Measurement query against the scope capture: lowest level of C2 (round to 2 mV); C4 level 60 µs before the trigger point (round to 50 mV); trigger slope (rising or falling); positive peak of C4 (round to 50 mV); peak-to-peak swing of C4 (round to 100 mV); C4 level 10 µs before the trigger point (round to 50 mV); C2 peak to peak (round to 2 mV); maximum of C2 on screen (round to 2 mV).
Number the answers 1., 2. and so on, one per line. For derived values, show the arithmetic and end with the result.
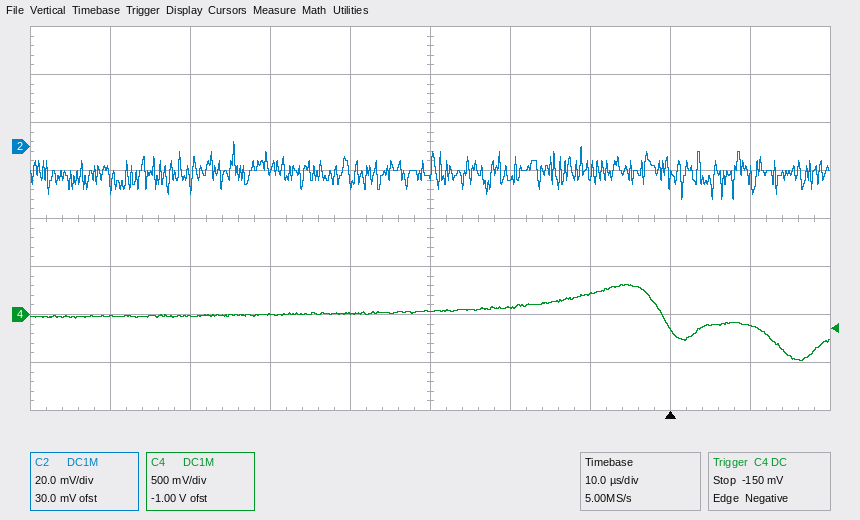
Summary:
1. -22 mV
2. 0 mV
3. falling
4. 300 mV
5. 800 mV
6. 200 mV
7. 2 mV − (-22 mV) = 24 mV
8. 2 mV
